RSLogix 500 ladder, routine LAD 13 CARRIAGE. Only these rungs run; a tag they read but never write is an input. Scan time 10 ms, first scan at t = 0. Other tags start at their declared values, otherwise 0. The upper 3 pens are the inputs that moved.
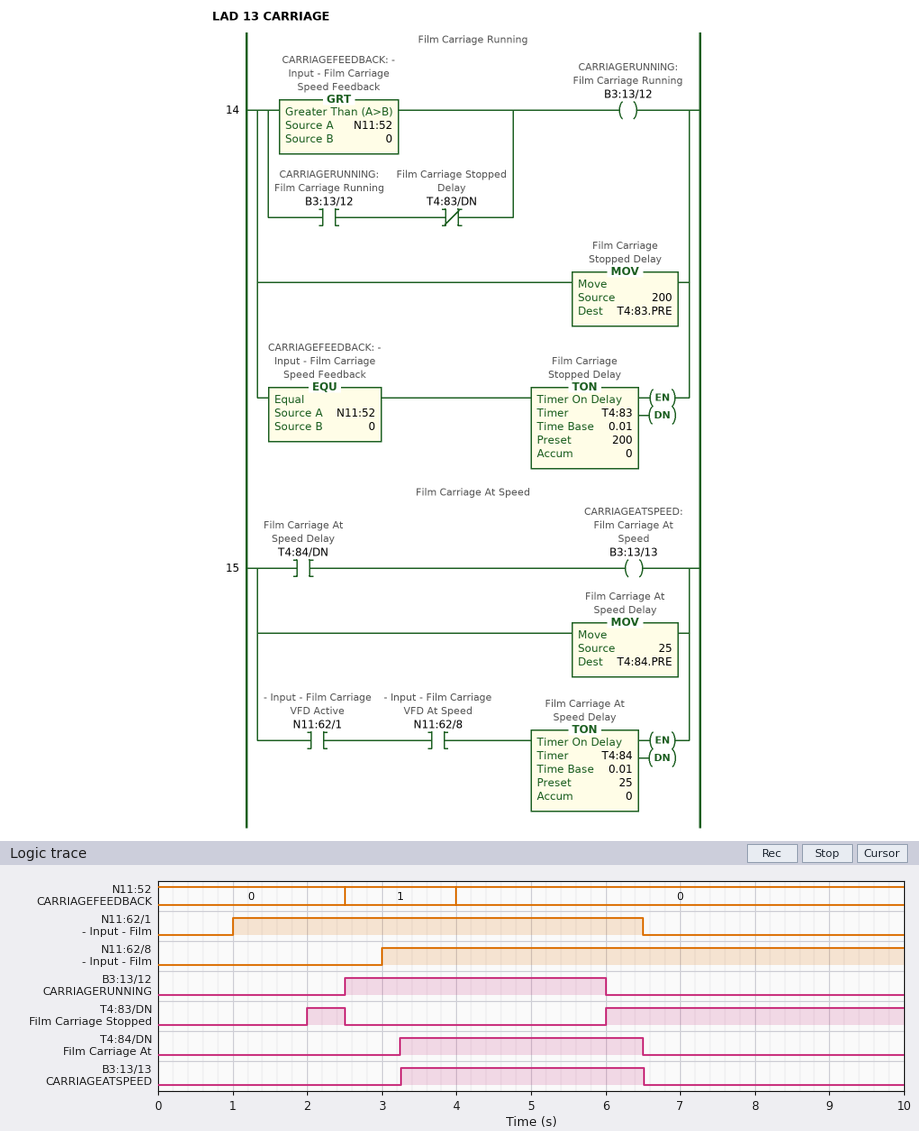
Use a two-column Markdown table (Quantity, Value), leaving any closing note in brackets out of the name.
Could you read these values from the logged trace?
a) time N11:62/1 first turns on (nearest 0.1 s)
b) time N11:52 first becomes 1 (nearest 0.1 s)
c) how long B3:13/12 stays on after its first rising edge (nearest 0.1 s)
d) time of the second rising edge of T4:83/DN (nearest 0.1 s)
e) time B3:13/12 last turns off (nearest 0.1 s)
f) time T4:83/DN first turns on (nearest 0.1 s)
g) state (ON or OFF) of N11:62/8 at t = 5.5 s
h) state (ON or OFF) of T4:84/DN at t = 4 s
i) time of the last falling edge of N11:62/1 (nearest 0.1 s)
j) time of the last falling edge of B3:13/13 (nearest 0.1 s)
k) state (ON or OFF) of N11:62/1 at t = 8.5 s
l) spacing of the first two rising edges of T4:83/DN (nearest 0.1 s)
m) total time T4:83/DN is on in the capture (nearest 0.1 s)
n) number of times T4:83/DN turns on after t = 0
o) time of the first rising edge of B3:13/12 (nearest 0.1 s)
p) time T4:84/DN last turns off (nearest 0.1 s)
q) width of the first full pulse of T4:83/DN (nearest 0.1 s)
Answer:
| Quantity | Value |
|---|---|
| time N11:62/1 first turns on | 1.0 s |
| time N11:52 first becomes 1 | 2.5 s |
| how long B3:13/12 stays on after its first rising edge | 3.5 s |
| time of the second rising edge of T4:83/DN | 6.0 s |
| time B3:13/12 last turns off | 6.0 s |
| time T4:83/DN first turns on | 2.0 s |
| state (ON or OFF) of N11:62/8 at t = 5.5 s | ON |
| state (ON or OFF) of T4:84/DN at t = 4 s | ON |
| time of the last falling edge of N11:62/1 | 6.5 s |
| time of the last falling edge of B3:13/13 | 6.5 s |
| state (ON or OFF) of N11:62/1 at t = 8.5 s | OFF |
| spacing of the first two rising edges of T4:83/DN | 4.0 s |
| total time T4:83/DN is on in the capture | 4.5 s |
| number of times T4:83/DN turns on after t = 0 | 2 |
| time of the first rising edge of B3:13/12 | 2.5 s |
| time T4:84/DN last turns off | 6.5 s |
| width of the first full pulse of T4:83/DN | 0.5 s |
